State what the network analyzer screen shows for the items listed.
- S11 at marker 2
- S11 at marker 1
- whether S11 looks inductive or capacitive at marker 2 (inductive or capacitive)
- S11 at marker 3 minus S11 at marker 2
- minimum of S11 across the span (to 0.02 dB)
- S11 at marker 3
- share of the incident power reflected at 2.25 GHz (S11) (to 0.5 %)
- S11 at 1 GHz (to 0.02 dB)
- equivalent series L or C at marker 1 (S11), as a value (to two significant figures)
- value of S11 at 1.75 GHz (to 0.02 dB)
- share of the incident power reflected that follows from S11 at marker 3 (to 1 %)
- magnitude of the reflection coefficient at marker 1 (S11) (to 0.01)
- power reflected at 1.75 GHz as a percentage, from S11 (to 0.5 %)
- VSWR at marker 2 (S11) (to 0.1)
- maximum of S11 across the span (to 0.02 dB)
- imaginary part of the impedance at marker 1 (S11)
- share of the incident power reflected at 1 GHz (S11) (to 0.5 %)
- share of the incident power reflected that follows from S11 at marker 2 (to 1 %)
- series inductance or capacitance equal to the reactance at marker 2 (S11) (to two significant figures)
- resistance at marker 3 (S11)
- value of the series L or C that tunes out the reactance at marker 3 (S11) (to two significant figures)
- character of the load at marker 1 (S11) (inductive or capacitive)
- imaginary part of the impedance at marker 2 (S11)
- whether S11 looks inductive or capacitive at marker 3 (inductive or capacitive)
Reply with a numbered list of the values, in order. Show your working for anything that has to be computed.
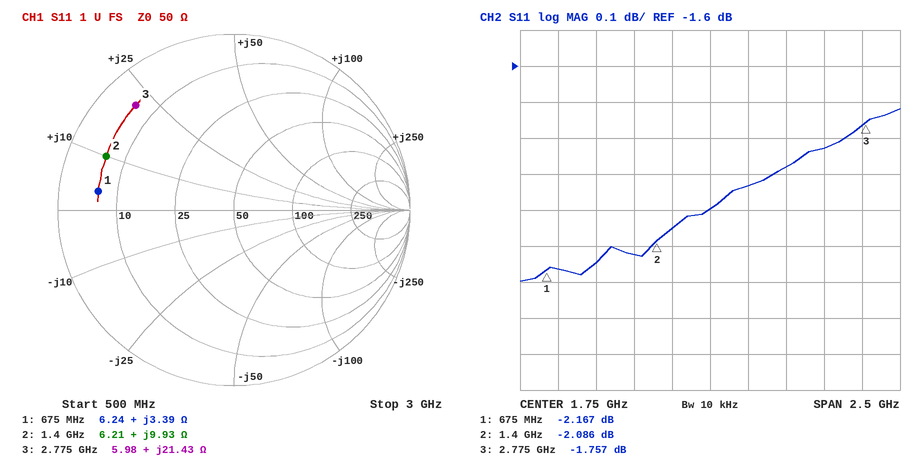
1. -2.086 dB
2. -2.167 dB
3. inductive
4. -1.757 − (-2.086) = 0.329 dB
5. -2.20 dB
6. -1.757 dB
7. 10^(-1.88/10) ≈ 64.9 %, so 65.0 % to the nearest 0.5 %
8. -2.14 dB
9. L = 3.39 Ω/(2π × 675 MHz) ≈ 799 pH, so 800 pH to two significant figures
10. -2.00 dB
11. 10^(-1.757/10) ≈ 67 %
12. 0.78
13. 10^(-2/10) ≈ 63.1 %, so 63.0 % to the nearest 0.5 %
14. 8.4
15. -1.72 dB
16. +3.39 Ω
17. 10^(-2.14/10) ≈ 61.1 %, so 61.0 % to the nearest 0.5 %
18. 10^(-2.086/10) ≈ 62 %
19. L = 9.93 Ω/(2π × 1.4 GHz) ≈ 1.1 nH
20. 5.98 Ω
21. C = 1/(2π × 2.775 GHz × 21.43 Ω) ≈ 2.7 pF
22. inductive
23. +9.93 Ω
24. inductive
